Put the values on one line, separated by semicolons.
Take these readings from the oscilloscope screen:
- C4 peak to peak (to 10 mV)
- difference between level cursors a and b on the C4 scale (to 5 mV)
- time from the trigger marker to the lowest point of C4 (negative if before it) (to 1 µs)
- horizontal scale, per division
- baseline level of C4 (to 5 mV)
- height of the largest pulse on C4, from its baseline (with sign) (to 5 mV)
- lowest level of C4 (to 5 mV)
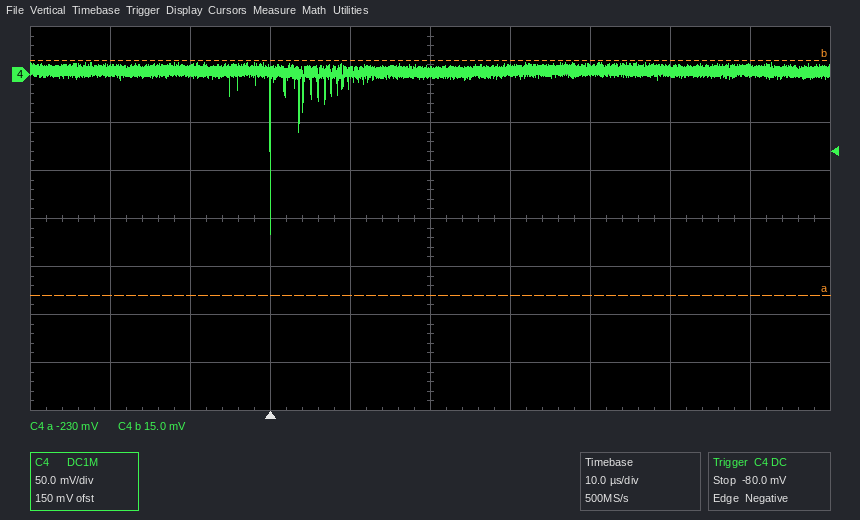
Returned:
180 mV; 245 mV; 0 µs; 10 µs; 5 mV; -170 mV; -165 mV
